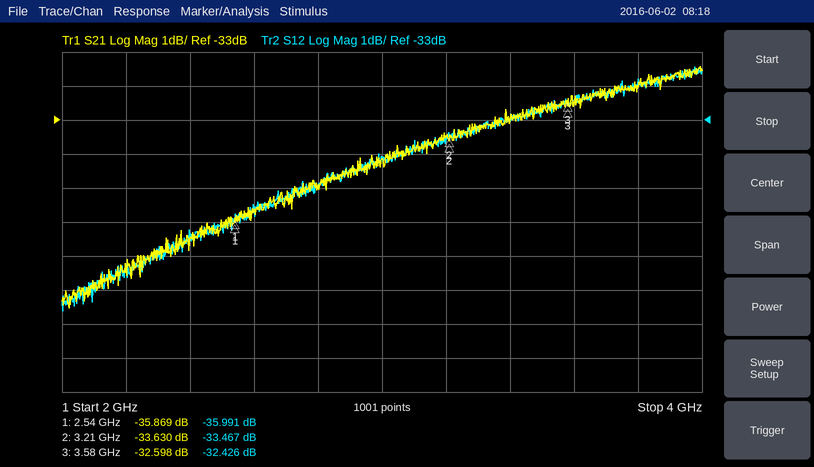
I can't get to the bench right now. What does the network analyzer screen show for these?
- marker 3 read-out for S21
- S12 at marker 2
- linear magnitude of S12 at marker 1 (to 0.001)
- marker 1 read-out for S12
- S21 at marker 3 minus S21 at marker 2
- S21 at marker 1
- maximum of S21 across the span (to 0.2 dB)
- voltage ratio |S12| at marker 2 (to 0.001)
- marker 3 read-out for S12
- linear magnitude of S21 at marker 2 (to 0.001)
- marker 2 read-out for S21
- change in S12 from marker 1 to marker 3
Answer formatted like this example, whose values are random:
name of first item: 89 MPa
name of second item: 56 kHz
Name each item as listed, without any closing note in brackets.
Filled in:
marker 3 read-out for S21: -32.598 dB
S12 at marker 2: -33.467 dB
linear magnitude of S12 at marker 1: 0.016
marker 1 read-out for S12: -35.991 dB
S21 at marker 3 minus S21 at marker 2: 1.032 dB
S21 at marker 1: -35.869 dB
maximum of S21 across the span: -31.4 dB
voltage ratio |S12| at marker 2: 0.021
marker 3 read-out for S12: -32.426 dB
linear magnitude of S21 at marker 2: 0.021
marker 2 read-out for S21: -33.630 dB
change in S12 from marker 1 to marker 3: 3.565 dB
